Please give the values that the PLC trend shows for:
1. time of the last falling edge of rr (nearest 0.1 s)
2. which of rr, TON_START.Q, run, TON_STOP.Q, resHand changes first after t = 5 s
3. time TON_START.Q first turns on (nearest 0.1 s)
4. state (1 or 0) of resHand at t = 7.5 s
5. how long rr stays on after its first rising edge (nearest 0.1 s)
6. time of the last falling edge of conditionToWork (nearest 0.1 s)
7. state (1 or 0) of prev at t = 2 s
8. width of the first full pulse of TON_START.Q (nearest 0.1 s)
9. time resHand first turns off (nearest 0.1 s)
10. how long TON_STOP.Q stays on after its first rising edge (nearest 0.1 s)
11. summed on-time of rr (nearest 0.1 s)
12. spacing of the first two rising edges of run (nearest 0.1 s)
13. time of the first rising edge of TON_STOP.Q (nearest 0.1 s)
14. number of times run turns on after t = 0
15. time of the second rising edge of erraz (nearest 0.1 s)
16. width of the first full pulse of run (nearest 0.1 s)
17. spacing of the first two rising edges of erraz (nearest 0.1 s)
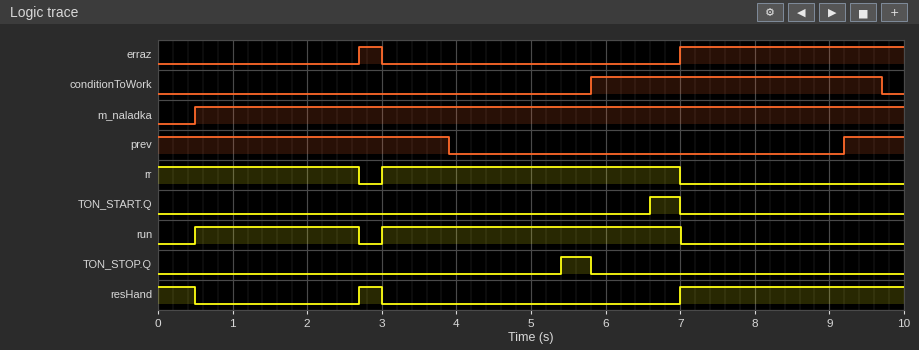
7.0 s
TON_STOP.Q
6.6 s
1
4.0 s
9.7 s
1
0.4 s
0.5 s
0.4 s
6.7 s
2.5 s
5.4 s
2
7.0 s
2.2 s
4.3 s
